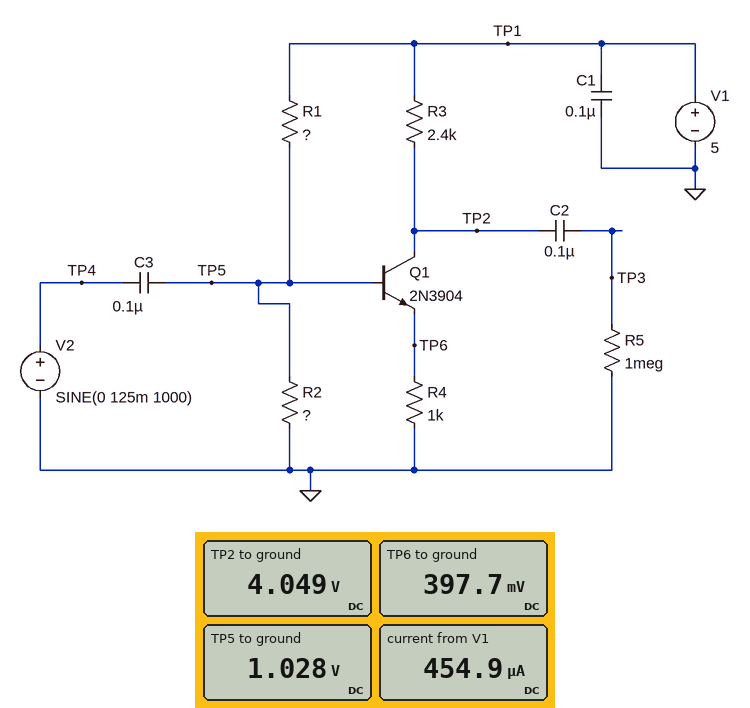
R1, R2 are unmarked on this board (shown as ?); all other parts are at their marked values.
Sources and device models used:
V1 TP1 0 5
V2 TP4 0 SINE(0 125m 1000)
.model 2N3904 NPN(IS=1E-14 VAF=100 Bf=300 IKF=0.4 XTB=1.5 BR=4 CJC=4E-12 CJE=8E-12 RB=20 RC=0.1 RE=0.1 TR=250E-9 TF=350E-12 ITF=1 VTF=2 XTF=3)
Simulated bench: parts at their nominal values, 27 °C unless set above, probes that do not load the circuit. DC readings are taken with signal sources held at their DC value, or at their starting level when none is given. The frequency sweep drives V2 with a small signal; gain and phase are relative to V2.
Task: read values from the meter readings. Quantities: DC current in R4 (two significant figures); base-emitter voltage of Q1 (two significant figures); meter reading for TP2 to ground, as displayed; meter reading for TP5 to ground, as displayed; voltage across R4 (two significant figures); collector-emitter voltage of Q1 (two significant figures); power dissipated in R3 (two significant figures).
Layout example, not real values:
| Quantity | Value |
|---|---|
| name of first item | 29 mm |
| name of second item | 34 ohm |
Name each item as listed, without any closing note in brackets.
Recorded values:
| Quantity | Value |
|---|---|
| DC current in R4 | 400 µA |
| base-emitter voltage of Q1 | 630 mV |
| meter reading for TP2 to ground, as displayed | 4.049 V |
| meter reading for TP5 to ground, as displayed | 1.028 V |
| voltage across R4 | 400 mV |
| collector-emitter voltage of Q1 | 3.7 V |
| power dissipated in R3 | 380 µW |
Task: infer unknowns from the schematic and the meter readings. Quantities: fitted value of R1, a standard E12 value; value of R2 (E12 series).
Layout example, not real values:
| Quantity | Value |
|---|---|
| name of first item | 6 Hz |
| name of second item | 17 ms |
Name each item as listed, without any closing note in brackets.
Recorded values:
| Quantity | Value |
|---|---|
| fitted value of R1, a standard E12 value | 68 kΩ |
| value of R2 | 18 kΩ |
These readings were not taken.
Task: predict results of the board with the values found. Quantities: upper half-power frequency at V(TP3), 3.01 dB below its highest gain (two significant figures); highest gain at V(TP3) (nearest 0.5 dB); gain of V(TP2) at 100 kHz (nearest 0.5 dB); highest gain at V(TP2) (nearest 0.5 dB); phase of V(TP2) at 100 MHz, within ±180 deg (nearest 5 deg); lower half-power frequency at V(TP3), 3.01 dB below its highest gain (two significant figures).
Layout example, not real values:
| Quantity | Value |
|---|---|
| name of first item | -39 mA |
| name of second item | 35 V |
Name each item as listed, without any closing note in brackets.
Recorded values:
| Quantity | Value |
|---|---|
| upper half-power frequency at V(TP3), 3.01 dB below its highest gain | 44 MHz |
| highest gain at V(TP3) | 7.0 dB |
| gain of V(TP2) at 100 kHz | 7.0 dB |
| highest gain at V(TP2) | 7.0 dB |
| phase of V(TP2) at 100 MHz, within ±180 deg | 35 deg |
| lower half-power frequency at V(TP3), 3.01 dB below its highest gain | 120 Hz |
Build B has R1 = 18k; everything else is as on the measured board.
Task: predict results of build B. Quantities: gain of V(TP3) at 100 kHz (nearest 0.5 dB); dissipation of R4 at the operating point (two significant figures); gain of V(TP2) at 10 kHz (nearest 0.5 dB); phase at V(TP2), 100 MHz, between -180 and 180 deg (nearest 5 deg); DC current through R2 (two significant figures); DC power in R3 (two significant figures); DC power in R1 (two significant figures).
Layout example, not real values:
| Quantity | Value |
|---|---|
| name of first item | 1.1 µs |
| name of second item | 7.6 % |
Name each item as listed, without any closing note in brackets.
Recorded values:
| Quantity | Value |
|---|---|
| gain of V(TP3) at 100 kHz | -7.0 dB |
| dissipation of R4 at the operating point | 2.2 mW |
| gain of V(TP2) at 10 kHz | -13.0 dB |
| phase at V(TP2), 100 MHz, between -180 and 180 deg | 0 deg |
| DC current through R2 | 120 µA |
| DC power in R3 | 5.0 mW |
| DC power in R1 | 450 µW |
